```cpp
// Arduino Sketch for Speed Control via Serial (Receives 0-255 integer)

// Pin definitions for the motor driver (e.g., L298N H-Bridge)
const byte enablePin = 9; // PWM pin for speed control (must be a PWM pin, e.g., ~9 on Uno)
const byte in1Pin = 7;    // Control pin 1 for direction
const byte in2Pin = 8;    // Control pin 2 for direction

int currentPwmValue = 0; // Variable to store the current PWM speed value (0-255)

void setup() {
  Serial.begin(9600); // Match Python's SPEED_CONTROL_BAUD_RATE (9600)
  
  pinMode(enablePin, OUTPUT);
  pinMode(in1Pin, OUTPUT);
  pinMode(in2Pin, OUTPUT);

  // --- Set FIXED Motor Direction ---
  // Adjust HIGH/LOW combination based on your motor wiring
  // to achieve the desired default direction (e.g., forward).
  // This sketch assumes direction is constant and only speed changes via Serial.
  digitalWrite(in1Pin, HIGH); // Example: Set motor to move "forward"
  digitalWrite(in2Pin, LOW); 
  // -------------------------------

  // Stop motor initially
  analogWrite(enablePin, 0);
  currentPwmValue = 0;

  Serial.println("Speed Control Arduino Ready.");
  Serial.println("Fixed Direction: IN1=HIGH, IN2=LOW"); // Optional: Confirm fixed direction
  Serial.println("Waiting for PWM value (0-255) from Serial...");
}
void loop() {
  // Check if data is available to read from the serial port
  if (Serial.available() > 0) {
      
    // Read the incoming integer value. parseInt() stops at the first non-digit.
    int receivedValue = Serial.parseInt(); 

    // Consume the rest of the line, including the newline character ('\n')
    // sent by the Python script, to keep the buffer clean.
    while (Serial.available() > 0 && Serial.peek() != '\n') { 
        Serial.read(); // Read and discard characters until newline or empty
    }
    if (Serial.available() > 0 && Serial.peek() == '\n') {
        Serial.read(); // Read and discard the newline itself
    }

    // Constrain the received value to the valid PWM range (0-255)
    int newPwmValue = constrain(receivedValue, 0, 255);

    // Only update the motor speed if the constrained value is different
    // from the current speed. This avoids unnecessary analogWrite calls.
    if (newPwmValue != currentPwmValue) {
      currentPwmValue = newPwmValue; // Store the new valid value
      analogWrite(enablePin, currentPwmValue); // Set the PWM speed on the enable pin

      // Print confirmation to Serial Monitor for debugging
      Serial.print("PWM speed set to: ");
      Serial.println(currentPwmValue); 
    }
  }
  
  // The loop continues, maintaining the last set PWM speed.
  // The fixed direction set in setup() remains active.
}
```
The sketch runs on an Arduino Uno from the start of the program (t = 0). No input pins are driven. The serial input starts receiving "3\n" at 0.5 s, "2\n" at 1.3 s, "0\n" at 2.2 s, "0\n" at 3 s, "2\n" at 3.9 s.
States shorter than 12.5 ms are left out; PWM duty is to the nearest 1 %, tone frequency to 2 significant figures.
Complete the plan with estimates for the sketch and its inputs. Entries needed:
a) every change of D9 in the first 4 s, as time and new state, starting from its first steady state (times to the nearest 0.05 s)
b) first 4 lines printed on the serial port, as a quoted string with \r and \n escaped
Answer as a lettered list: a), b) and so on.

a) 0 s low; 0.5 s PWM 1 %; 1.3 s PWM 1 %; 2.2 s low; 3.9 s PWM 1 %
b) "Speed Control Arduino Ready.\r\nFixed Direction: IN1=HIGH, IN2=LOW\r\nWaiting for PWM value (0-255) from Serial...\r\nPWM speed set to: 3\r\n"
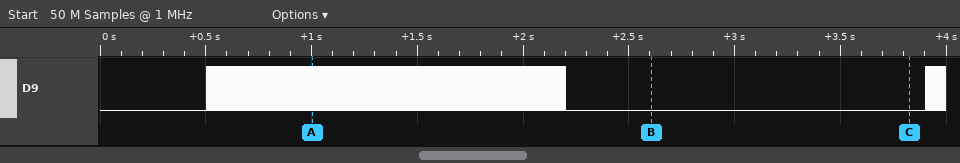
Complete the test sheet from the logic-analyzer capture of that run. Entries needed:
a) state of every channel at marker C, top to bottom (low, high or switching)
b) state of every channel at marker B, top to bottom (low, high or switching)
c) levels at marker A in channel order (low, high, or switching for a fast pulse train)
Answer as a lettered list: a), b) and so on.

a) D9 low
b) D9 low
c) D9 switching
